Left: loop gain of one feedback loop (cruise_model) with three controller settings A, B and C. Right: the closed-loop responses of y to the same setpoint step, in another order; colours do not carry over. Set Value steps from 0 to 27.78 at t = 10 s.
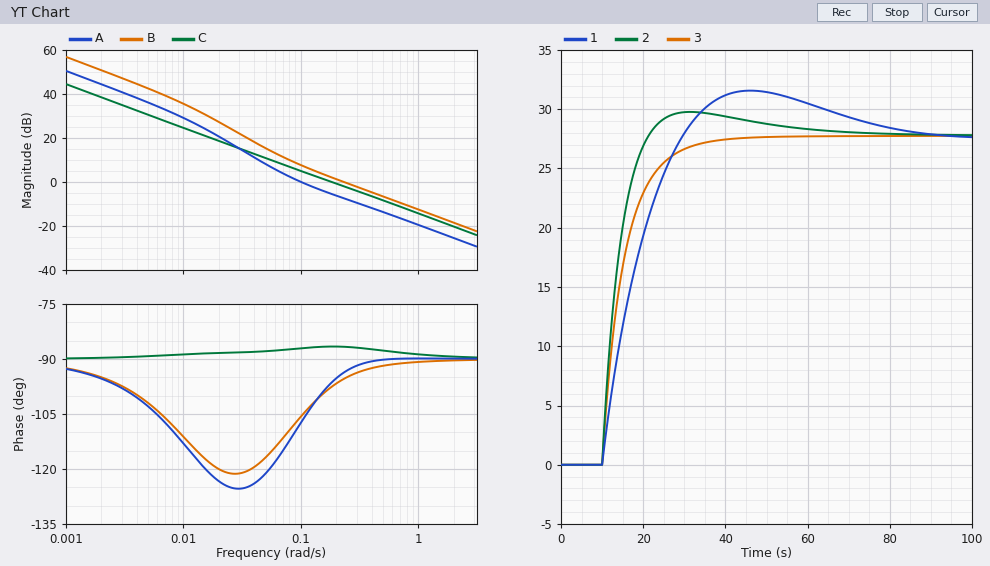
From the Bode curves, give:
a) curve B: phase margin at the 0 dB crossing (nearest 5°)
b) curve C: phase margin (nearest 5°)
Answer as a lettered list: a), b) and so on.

a) 85°
b) 95°
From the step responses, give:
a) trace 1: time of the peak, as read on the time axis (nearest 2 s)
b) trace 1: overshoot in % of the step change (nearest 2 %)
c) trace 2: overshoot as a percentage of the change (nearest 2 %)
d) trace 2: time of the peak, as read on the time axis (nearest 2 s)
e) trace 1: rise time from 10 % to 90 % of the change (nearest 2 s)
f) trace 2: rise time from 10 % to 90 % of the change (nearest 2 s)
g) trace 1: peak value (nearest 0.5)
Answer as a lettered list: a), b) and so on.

a) 46 s
b) 14 %
c) 8 %
d) 32 s
e) 14 s
f) 8 s
g) 31.5
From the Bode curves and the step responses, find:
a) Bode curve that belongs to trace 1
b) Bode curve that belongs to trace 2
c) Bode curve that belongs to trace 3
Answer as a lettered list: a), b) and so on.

a) A
b) B
c) C
